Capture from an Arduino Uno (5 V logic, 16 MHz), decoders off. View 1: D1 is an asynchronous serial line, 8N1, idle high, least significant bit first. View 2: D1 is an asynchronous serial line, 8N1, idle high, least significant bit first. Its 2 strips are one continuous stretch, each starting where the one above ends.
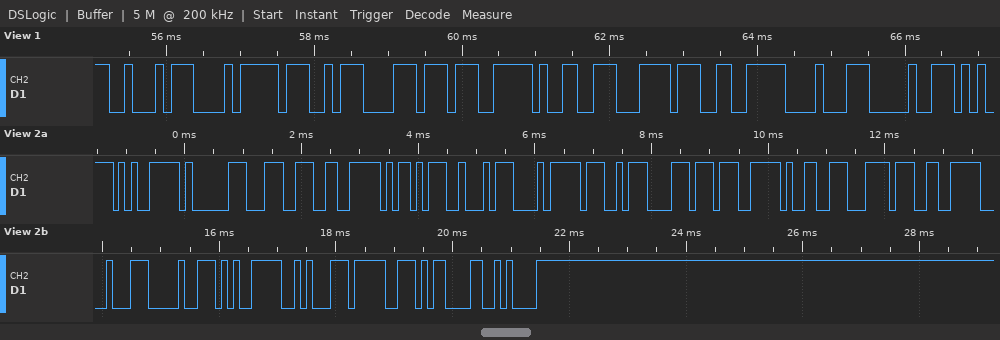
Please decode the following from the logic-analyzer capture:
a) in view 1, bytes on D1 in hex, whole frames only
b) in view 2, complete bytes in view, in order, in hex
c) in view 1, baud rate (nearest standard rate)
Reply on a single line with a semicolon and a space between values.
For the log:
A2 E8 A7 B8 E7 99 BC E6 88 90; 0xE5 0x81 0x9C 0xE6 0xAD 0xA2 0xE8 0xA7 0xB8 0xE7 0x99 0xBC 0xE6 0x88 0x90 0xE5 0x8A 0x9F 0x0D 0x0A; 9600 baud
